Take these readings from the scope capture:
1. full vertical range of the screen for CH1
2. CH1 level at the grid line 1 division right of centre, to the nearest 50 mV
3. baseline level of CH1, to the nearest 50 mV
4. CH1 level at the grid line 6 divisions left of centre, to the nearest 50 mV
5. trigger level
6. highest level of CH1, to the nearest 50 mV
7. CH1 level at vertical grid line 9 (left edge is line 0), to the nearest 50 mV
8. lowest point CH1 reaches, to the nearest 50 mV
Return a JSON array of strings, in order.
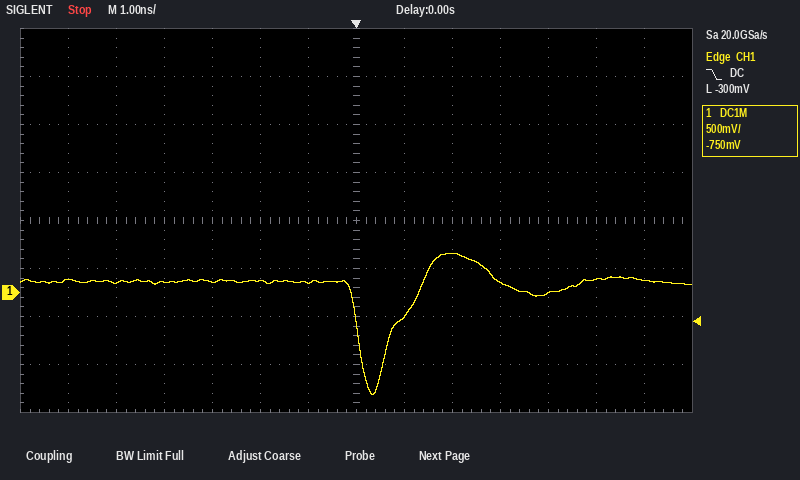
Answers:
["4 V", "-250 mV", "100 mV", "150 mV", "-300 mV", "400 mV", "400 mV", "-1.05 V"]
